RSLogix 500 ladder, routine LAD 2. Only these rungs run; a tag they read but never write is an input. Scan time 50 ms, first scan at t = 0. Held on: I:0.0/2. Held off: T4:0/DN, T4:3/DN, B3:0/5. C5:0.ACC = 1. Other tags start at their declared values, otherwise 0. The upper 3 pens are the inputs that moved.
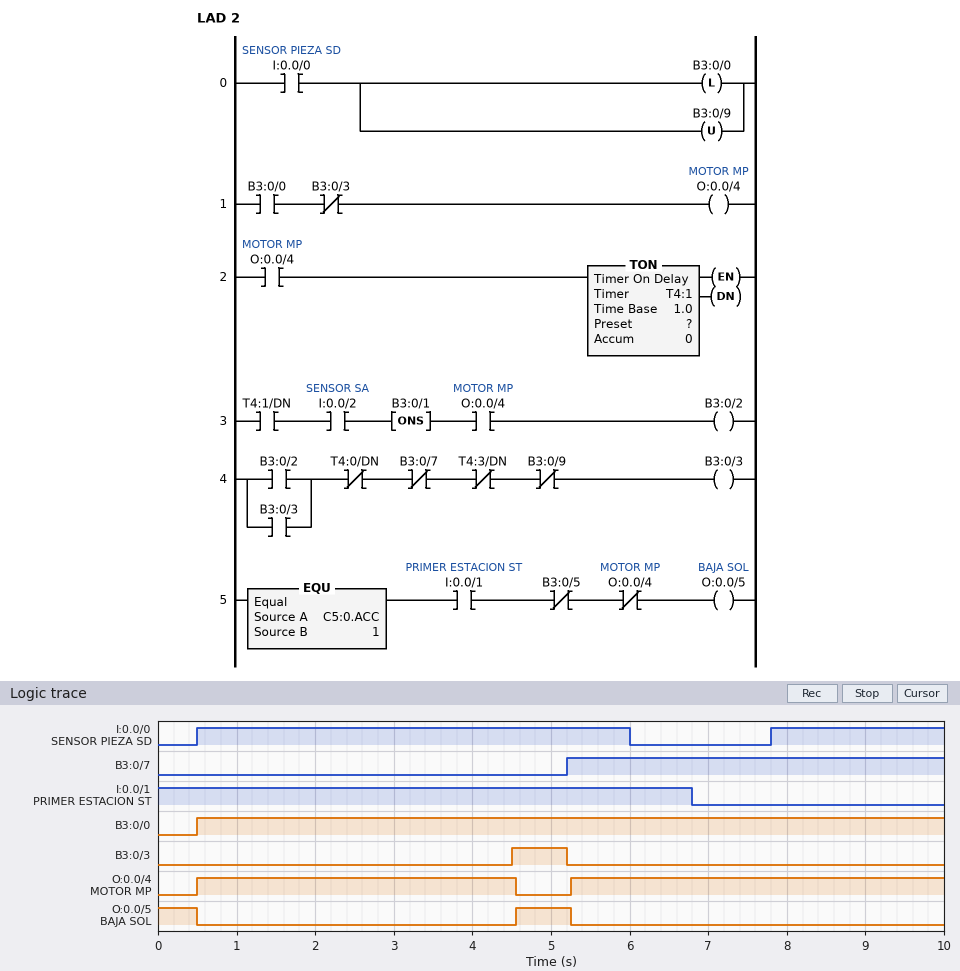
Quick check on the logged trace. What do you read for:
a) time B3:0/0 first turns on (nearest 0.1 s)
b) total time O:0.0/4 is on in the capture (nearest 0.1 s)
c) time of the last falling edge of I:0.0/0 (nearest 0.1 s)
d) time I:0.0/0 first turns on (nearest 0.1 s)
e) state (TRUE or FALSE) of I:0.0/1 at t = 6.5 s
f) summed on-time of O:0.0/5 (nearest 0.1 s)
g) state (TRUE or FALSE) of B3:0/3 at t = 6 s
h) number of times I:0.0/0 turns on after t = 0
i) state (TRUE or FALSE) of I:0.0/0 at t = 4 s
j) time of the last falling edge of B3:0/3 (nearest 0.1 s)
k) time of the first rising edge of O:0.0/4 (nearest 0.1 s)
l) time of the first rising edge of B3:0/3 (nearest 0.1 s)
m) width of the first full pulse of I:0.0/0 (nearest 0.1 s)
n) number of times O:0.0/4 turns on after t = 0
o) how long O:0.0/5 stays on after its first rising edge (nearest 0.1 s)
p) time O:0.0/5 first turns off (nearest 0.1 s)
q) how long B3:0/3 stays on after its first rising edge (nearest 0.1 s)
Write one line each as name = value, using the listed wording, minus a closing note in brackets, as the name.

time B3:0/0 first turns on = 0.5 s
total time O:0.0/4 is on in the capture = 8.8 s
time of the last falling edge of I:0.0/0 = 6.0 s
time I:0.0/0 first turns on = 0.5 s
state (TRUE or FALSE) of I:0.0/1 at t = 6.5 s = TRUE
summed on-time of O:0.0/5 = 1.2 s
state (TRUE or FALSE) of B3:0/3 at t = 6 s = FALSE
number of times I:0.0/0 turns on after t = 0 = 2
state (TRUE or FALSE) of I:0.0/0 at t = 4 s = TRUE
time of the last falling edge of B3:0/3 = 5.2 s
time of the first rising edge of O:0.0/4 = 0.5 s
time of the first rising edge of B3:0/3 = 4.5 s
width of the first full pulse of I:0.0/0 = 5.5 s
number of times O:0.0/4 turns on after t = 0 = 2
how long O:0.0/5 stays on after its first rising edge = 0.7 s
time O:0.0/5 first turns off = 0.5 s
how long B3:0/3 stays on after its first rising edge = 0.7 s
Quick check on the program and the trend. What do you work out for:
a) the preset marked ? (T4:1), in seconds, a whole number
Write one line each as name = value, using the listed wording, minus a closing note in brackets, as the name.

the preset marked ? (T4:1), in seconds, a whole number = 4 s
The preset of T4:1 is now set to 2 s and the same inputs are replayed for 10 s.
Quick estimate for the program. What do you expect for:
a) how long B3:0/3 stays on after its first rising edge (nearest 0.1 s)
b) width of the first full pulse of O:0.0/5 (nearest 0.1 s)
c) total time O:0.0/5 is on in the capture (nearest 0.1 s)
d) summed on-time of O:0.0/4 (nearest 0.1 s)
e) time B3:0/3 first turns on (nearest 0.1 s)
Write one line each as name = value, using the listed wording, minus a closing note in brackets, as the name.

how long B3:0/3 stays on after its first rising edge = 2.7 s
width of the first full pulse of O:0.0/5 = 2.7 s
total time O:0.0/5 is on in the capture = 3.2 s
summed on-time of O:0.0/4 = 6.8 s
time B3:0/3 first turns on = 2.5 s
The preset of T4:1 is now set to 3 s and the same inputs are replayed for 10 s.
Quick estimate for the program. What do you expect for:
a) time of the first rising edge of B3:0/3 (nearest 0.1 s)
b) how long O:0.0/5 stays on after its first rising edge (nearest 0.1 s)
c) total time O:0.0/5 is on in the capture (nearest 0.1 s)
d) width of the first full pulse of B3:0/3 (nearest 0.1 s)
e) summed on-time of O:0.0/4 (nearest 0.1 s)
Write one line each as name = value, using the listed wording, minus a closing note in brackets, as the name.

time of the first rising edge of B3:0/3 = 3.5 s
how long O:0.0/5 stays on after its first rising edge = 1.7 s
total time O:0.0/5 is on in the capture = 2.2 s
width of the first full pulse of B3:0/3 = 1.7 s
summed on-time of O:0.0/4 = 7.8 s
